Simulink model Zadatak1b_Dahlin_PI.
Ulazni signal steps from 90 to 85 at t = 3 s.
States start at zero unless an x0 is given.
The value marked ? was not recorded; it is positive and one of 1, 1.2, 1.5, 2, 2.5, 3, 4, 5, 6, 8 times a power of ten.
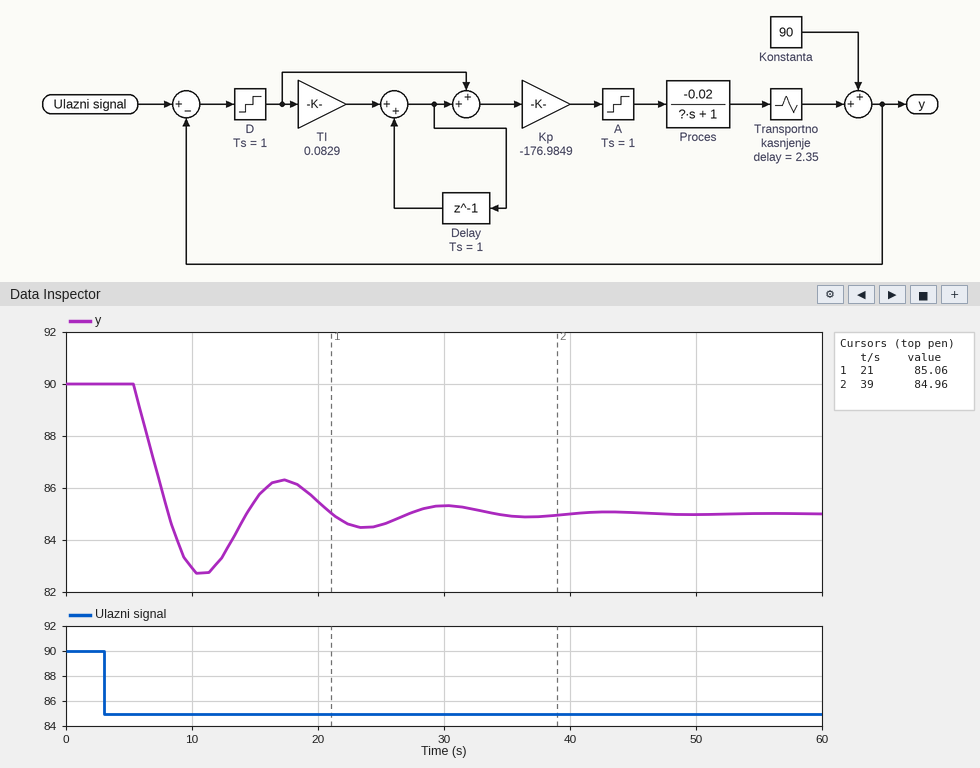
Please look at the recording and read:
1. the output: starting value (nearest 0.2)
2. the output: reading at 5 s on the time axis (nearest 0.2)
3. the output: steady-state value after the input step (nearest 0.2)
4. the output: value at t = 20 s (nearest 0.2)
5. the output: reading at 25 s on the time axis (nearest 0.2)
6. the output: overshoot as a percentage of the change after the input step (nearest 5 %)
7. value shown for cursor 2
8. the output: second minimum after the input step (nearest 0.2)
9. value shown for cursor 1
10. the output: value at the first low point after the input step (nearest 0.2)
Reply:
90.0
90.0
85.0
85.4
84.6
45 %
84.96
84.4
85.06
82.8
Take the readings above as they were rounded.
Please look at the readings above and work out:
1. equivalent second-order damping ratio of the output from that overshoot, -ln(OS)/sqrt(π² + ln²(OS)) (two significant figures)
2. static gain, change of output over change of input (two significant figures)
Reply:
0.25
1.0
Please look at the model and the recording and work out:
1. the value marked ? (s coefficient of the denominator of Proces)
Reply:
10
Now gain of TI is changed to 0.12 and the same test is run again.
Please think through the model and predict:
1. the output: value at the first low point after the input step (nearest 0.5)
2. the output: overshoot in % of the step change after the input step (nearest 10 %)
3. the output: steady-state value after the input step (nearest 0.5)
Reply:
82.0
60 %
85.0
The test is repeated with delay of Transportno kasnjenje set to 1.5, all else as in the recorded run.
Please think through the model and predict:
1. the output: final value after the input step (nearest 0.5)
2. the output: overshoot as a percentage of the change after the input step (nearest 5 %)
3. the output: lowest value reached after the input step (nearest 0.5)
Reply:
85.0
20 %
84.0
